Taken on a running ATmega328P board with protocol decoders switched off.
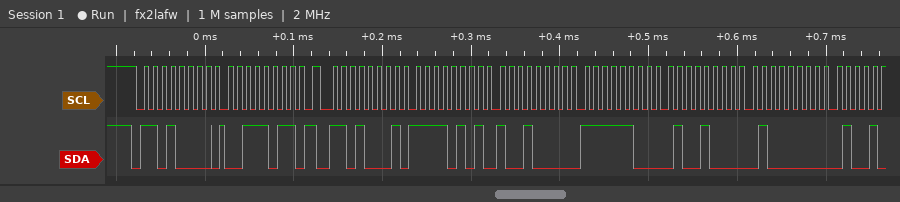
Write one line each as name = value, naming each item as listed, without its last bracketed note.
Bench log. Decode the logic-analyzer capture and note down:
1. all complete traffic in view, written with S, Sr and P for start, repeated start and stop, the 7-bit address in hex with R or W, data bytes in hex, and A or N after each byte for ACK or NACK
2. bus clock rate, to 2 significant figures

all complete traffic in view, written with S, Sr and P for start, repeated start and stop, the 7-bit address in hex with R or W, data bytes in hex, and A or N after each byte for ACK or NACK = S 68W A 3B A Sr 68R A F5 A 90 A FC A 48 A 40 A
bus clock rate, to 2 significant figures = 100 kHz
